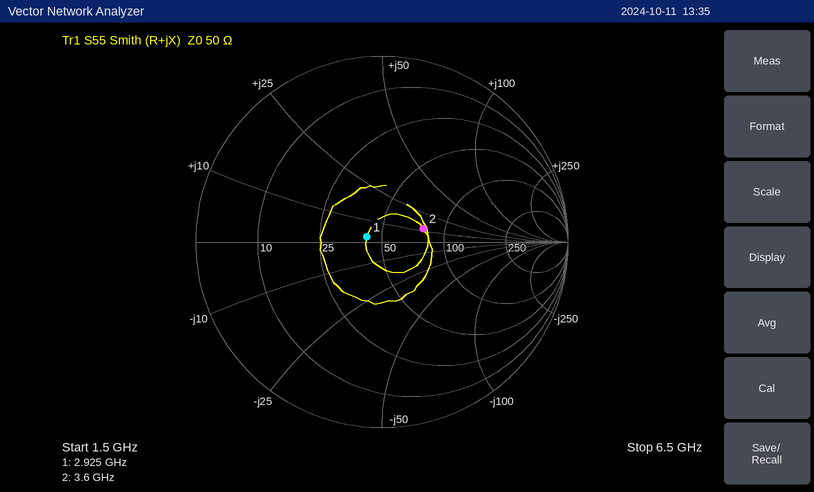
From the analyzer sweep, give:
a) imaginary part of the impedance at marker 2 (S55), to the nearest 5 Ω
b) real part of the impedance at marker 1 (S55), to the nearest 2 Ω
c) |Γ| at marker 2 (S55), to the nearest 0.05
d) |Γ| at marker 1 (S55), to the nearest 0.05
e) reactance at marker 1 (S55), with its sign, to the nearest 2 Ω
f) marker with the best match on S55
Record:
+10 Ω
42 Ω
0.25
0.10
+2 Ω
marker 1
